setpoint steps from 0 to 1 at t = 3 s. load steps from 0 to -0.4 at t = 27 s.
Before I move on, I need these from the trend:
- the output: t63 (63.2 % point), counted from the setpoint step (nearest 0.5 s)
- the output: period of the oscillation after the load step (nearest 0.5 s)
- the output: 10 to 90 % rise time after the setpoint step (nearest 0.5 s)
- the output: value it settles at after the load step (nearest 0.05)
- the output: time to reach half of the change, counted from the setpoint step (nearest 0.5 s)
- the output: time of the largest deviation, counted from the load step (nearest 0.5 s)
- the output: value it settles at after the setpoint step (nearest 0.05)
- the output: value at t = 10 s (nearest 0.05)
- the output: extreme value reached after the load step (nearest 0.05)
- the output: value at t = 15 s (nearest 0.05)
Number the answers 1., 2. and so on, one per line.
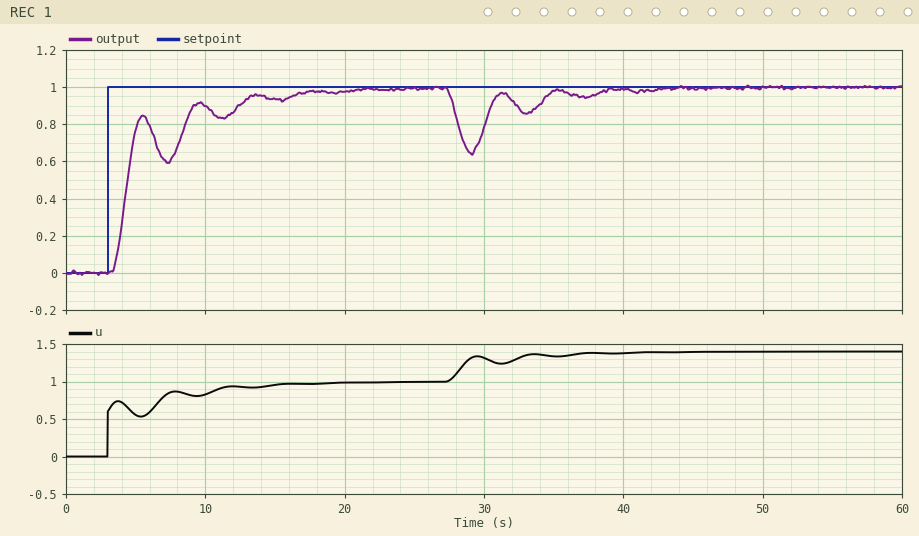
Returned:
1. 1.5 s
2. 4.0 s
3. 5.5 s
4. 1.00
5. 1.5 s
6. 2.0 s
7. 1.00
8. 0.90
9. 0.65
10. 0.95
